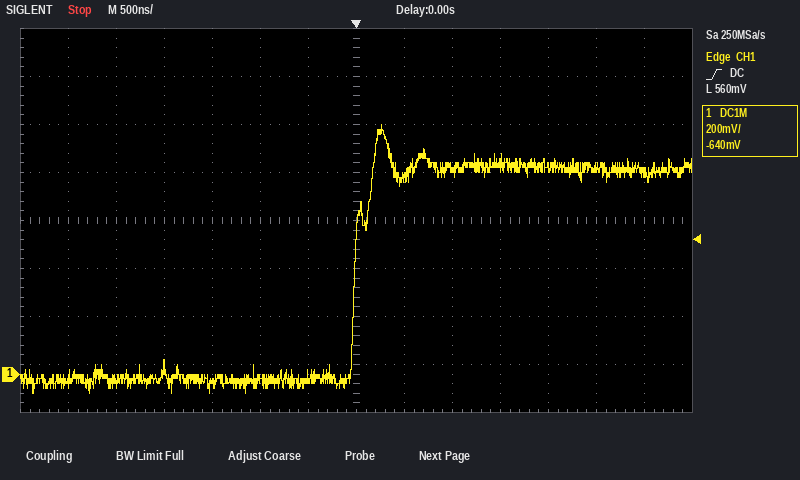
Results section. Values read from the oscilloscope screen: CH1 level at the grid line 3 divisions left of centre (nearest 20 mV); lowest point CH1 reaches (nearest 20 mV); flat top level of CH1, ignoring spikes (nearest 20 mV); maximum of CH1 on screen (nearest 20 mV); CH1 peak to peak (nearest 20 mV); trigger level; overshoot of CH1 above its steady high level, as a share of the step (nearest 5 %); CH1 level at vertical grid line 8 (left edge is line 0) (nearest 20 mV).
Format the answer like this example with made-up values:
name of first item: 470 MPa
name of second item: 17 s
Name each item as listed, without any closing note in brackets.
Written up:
CH1 level at the grid line 3 divisions left of centre: -40 mV
lowest point CH1 reaches: -80 mV
flat top level of CH1, ignoring spikes: 860 mV
maximum of CH1 on screen: 1.04 V
CH1 peak to peak: 1.12 V
trigger level: 560 mV
overshoot of CH1 above its steady high level, as a share of the step: 20 %
CH1 level at vertical grid line 8 (left edge is line 0): 820 mV
